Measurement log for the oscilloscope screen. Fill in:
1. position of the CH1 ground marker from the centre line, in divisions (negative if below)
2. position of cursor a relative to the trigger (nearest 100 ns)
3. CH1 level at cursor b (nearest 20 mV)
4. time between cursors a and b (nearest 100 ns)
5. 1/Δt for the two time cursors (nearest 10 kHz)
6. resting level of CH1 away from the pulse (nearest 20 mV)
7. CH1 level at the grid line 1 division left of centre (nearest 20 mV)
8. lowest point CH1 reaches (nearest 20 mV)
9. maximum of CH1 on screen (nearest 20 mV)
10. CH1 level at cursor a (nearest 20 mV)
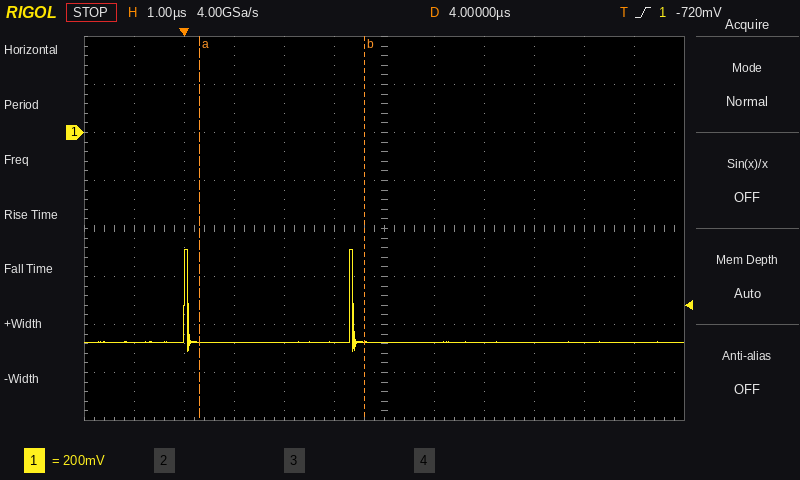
+2.0 div
+300 ns
-880 mV
3.3 µs
300 kHz
-880 mV
-880 mV
-920 mV
-480 mV
-880 mV
